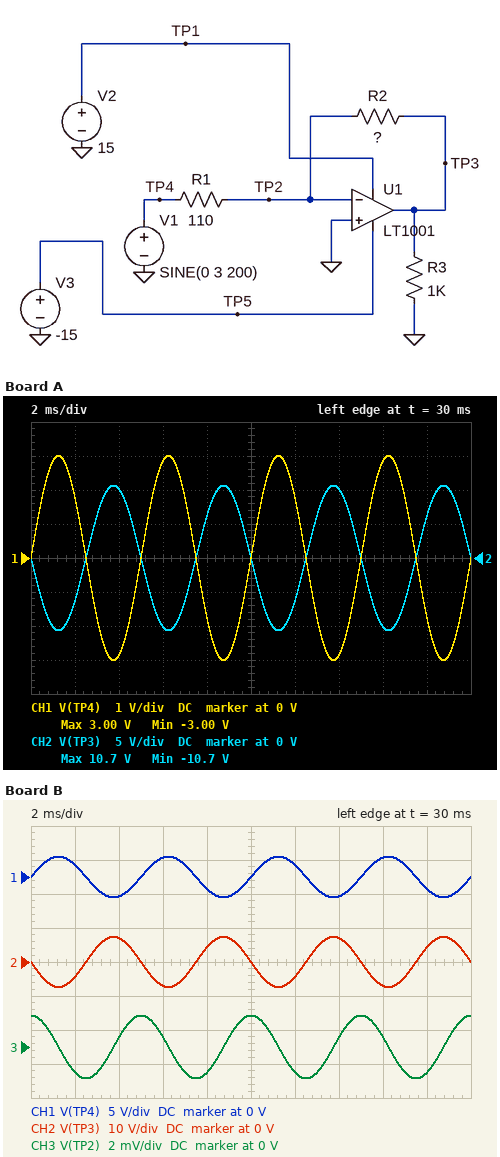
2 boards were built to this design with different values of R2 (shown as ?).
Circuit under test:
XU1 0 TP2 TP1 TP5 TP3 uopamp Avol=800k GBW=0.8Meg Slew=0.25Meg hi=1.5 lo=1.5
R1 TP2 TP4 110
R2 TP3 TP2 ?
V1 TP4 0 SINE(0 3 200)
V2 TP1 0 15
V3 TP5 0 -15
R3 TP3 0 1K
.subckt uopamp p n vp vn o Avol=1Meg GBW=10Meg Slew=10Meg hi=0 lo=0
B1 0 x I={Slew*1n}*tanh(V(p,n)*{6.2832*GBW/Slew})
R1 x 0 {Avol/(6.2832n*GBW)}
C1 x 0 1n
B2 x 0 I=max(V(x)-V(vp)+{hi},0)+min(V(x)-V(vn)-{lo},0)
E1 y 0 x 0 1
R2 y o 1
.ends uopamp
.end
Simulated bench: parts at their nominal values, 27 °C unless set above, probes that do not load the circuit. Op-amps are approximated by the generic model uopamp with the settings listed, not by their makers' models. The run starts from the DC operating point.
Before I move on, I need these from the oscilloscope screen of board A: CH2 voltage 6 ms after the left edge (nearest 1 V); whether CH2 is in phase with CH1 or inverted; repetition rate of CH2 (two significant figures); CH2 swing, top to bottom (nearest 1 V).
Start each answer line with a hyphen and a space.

- -10 V
- inverted
- 200 Hz
- 21 V
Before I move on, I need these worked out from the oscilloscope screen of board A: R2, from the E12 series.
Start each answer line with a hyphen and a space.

- 390 Ω
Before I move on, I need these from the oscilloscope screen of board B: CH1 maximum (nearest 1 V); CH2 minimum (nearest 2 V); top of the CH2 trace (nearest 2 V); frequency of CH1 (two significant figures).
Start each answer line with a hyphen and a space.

- 3 V
- -8 V
- 8 V
- 200 Hz
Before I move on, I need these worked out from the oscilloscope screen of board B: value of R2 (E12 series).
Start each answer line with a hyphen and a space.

- 270 Ω
